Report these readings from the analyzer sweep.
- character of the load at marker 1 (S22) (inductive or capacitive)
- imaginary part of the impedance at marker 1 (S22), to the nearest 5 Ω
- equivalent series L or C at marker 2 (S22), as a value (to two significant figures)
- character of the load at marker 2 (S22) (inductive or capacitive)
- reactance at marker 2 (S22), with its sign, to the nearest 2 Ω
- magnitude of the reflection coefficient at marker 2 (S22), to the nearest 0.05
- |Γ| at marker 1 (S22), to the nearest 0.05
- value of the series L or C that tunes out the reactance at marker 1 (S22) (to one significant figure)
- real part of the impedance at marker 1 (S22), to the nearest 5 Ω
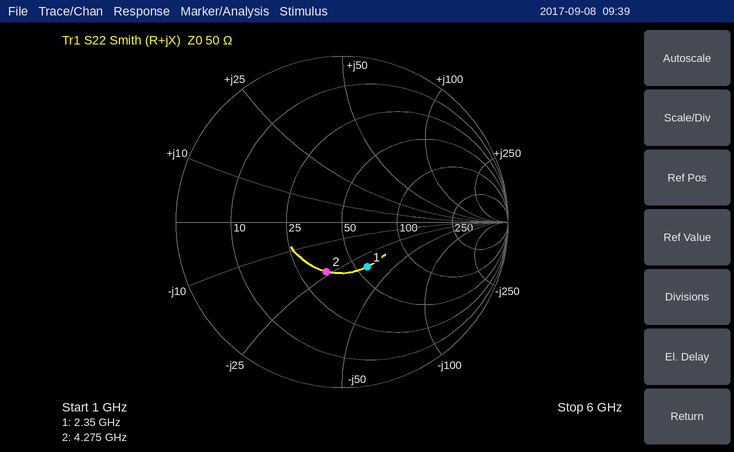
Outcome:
capacitive
-35 Ω
1.6 pF
capacitive
-24 Ω
0.30
0.30
2 nH
55 Ω
